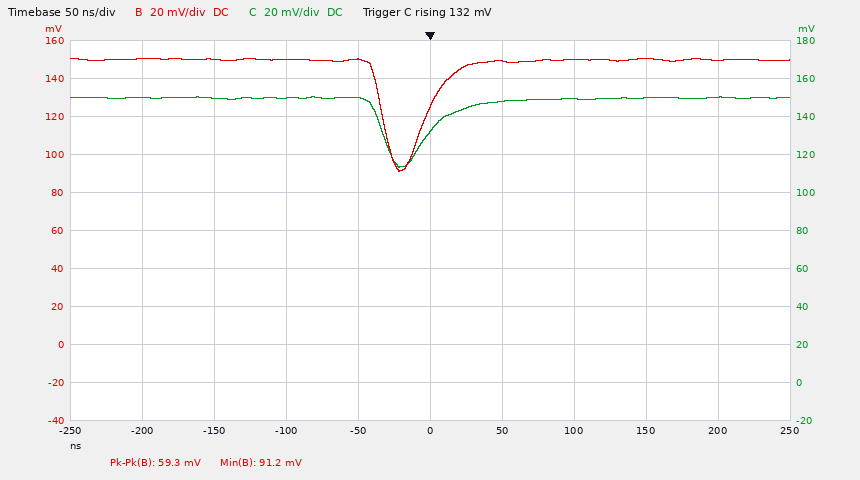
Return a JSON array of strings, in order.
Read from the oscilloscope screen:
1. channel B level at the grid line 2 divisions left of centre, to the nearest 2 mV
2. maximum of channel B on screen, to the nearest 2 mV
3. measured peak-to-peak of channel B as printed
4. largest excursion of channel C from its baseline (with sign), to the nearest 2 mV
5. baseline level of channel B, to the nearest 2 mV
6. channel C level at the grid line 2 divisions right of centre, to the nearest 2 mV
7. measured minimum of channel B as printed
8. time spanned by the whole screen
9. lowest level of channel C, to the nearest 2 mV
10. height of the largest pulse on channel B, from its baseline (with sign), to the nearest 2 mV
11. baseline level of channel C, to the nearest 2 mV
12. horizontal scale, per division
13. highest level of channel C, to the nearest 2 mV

["150 mV", "150 mV", "59.3 mV", "-36 mV", "150 mV", "150 mV", "91.2 mV", "500 ns", "114 mV", "-58 mV", "150 mV", "50 ns", "150 mV"]
